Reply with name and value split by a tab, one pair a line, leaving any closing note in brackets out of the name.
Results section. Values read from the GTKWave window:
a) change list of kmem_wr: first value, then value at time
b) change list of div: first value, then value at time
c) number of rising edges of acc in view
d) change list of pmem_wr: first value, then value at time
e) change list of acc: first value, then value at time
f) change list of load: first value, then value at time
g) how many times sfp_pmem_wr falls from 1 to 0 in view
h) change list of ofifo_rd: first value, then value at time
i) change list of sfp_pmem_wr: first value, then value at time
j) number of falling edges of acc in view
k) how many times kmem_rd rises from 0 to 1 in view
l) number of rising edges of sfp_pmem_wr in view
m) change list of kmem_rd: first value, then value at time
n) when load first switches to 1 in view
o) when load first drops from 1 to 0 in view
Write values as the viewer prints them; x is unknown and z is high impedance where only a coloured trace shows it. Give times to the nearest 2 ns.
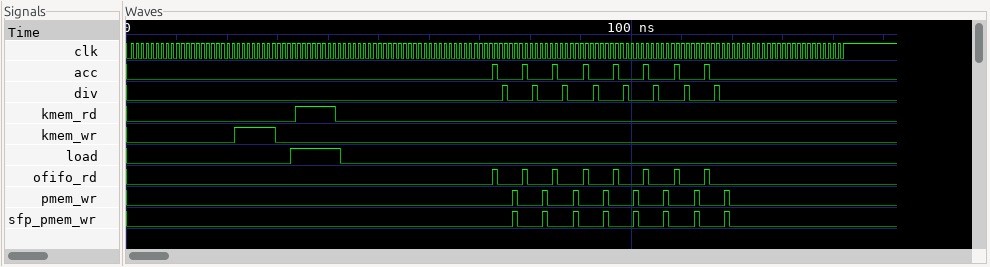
change list of kmem_wr: first value, then value at time	0, 1 at 22 ns, 0 at 30 ns
change list of div: first value, then value at time	0, 1 at 74 ns, 0 at 76 ns, 1 at 80 ns, 0 at 82 ns, 1 at 86 ns, 0 at 88 ns, 1 at 92 ns, 0 at 94 ns, 1 at 98 ns, 0 at 100 ns, 1 at 104 ns, 0 at 106 ns, 1 at 110 ns, 0 at 112 ns, 1 at 116 ns, 0 at 118 ns
number of rising edges of acc in view	8
change list of pmem_wr: first value, then value at time	0, 1 at 76 ns, 0 at 78 ns, 1 at 82 ns, 0 at 84 ns, 1 at 88 ns, 0 at 90 ns, 1 at 94 ns, 0 at 96 ns, 1 at 100 ns, 0 at 102 ns, 1 at 106 ns, 0 at 108 ns, 1 at 112 ns, 0 at 114 ns, 1 at 118 ns, 0 at 120 ns
change list of acc: first value, then value at time	0, 1 at 72 ns, 0 at 74 ns, 1 at 78 ns, 0 at 80 ns, 1 at 84 ns, 0 at 86 ns, 1 at 90 ns, 0 at 92 ns, 1 at 96 ns, 0 at 98 ns, 1 at 102 ns, 0 at 104 ns, 1 at 108 ns, 0 at 110 ns, 1 at 114 ns, 0 at 116 ns
change list of load: first value, then value at time	0, 1 at 32 ns, 0 at 42 ns
how many times sfp_pmem_wr falls from 1 to 0 in view	8
change list of ofifo_rd: first value, then value at time	0, 1 at 72 ns, 0 at 74 ns, 1 at 78 ns, 0 at 80 ns, 1 at 84 ns, 0 at 86 ns, 1 at 90 ns, 0 at 92 ns, 1 at 96 ns, 0 at 98 ns, 1 at 102 ns, 0 at 104 ns, 1 at 108 ns, 0 at 110 ns, 1 at 114 ns, 0 at 116 ns
change list of sfp_pmem_wr: first value, then value at time	0, 1 at 76 ns, 0 at 78 ns, 1 at 82 ns, 0 at 84 ns, 1 at 88 ns, 0 at 90 ns, 1 at 94 ns, 0 at 96 ns, 1 at 100 ns, 0 at 102 ns, 1 at 106 ns, 0 at 108 ns, 1 at 112 ns, 0 at 114 ns, 1 at 118 ns, 0 at 120 ns
number of falling edges of acc in view	8
how many times kmem_rd rises from 0 to 1 in view	1
number of rising edges of sfp_pmem_wr in view	8
change list of kmem_rd: first value, then value at time	0, 1 at 34 ns, 0 at 42 ns
when load first switches to 1 in view	32 ns
when load first drops from 1 to 0 in view	42 ns
